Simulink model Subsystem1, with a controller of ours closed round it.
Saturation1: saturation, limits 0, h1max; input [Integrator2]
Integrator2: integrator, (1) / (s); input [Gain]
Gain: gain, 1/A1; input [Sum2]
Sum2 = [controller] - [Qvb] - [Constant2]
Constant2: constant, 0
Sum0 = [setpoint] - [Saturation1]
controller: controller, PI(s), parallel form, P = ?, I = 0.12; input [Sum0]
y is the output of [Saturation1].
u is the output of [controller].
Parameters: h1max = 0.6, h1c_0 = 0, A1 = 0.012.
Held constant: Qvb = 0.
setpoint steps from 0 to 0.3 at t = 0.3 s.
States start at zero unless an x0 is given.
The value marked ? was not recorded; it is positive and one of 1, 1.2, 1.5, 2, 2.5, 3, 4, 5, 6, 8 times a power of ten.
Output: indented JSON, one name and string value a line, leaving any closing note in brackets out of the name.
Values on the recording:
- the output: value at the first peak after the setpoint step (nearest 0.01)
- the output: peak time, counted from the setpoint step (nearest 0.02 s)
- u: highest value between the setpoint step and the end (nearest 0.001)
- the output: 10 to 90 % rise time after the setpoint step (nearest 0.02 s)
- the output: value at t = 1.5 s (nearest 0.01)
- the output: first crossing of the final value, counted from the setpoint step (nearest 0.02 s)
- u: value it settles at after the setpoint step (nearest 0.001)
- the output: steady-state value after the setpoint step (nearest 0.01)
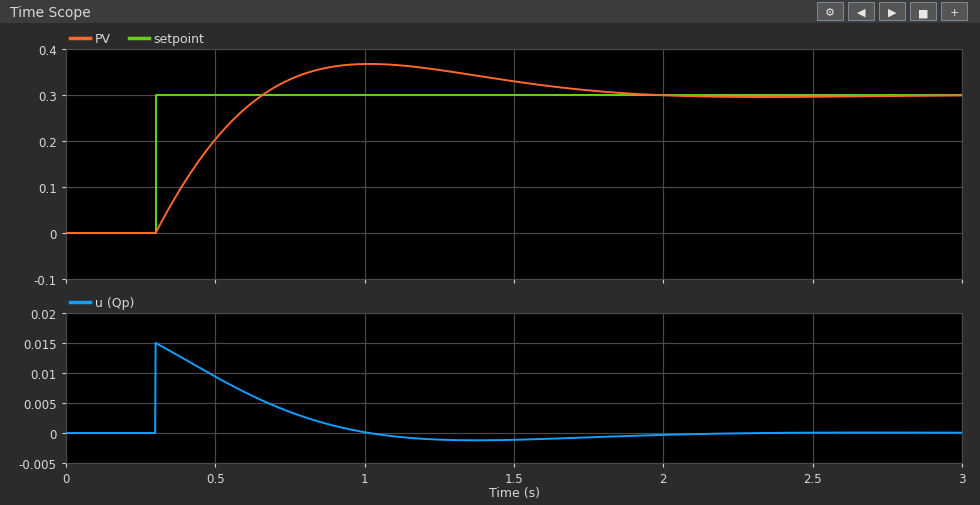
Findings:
{
  "the output: value at the first peak after the setpoint step": "0.37",
  "the output: peak time, counted from the setpoint step": "0.72 s",
  "u: highest value between the setpoint step and the end": "0.015",
  "the output: 10 to 90 % rise time after the setpoint step": "0.28 s",
  "the output: value at t = 1.5 s": "0.33",
  "the output: first crossing of the final value, counted from the setpoint step": "0.36 s",
  "u: value it settles at after the setpoint step": "0.000",
  "the output: steady-state value after the setpoint step": "0.30"
}
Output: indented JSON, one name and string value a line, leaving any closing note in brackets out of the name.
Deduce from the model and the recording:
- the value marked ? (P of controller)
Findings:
{
  "the value marked ?": "0.05"
}
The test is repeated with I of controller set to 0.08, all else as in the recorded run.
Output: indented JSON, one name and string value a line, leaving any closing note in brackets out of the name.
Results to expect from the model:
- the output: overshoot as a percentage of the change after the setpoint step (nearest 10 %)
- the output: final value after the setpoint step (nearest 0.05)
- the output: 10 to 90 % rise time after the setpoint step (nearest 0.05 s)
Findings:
{
  "the output: overshoot as a percentage of the change after the setpoint step": "20 %",
  "the output: final value after the setpoint step": "0.30",
  "the output: 10 to 90 % rise time after the setpoint step": "0.30 s"
}
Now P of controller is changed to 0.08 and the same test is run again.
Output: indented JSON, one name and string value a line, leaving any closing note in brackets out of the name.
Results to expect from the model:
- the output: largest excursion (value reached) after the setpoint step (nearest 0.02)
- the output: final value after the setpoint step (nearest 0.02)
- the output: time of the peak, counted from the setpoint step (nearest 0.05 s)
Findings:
{
  "the output: largest excursion (value reached) after the setpoint step": "0.34",
  "the output: final value after the setpoint step": "0.30",
  "the output: time of the peak, counted from the setpoint step": "0.60 s"
}
